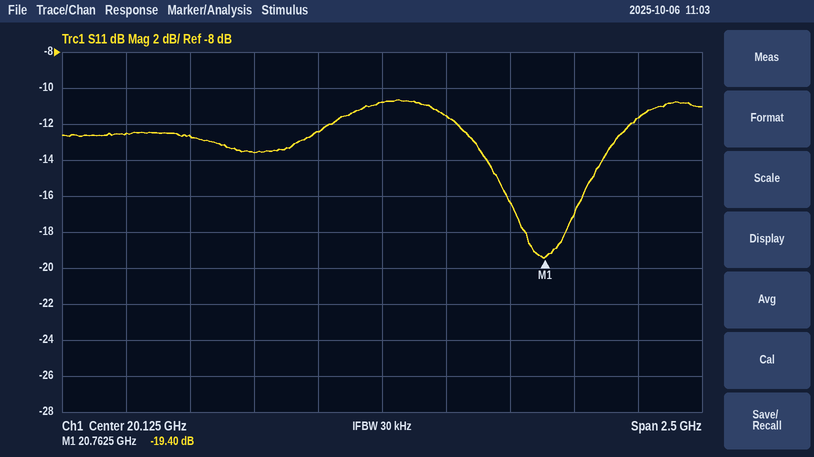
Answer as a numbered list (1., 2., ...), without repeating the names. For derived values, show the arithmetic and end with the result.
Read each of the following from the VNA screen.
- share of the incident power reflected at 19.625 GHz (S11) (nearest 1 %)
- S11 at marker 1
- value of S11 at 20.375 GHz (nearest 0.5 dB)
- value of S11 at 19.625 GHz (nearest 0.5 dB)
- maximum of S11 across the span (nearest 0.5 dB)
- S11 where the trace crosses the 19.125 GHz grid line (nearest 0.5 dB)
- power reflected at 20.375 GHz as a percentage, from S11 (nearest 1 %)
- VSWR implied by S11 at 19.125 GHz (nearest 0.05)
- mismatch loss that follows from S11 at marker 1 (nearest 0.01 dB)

1. 10^(-13.5/10) ≈ 4 %
2. -19.40 dB
3. -11.5 dB
4. -13.5 dB
5. -10.5 dB
6. -12.5 dB
7. 10^(-11.5/10) ≈ 7 %
8. |Γ| = 10^(-12.5/20) = 0.2371; VSWR = (1 + 0.2371)/(1 − 0.2371) ≈ 1.62, so 1.60 to the nearest 0.05
9. −10 log10(1 − 10^(-19.4/10)) ≈ 0.05 dB
